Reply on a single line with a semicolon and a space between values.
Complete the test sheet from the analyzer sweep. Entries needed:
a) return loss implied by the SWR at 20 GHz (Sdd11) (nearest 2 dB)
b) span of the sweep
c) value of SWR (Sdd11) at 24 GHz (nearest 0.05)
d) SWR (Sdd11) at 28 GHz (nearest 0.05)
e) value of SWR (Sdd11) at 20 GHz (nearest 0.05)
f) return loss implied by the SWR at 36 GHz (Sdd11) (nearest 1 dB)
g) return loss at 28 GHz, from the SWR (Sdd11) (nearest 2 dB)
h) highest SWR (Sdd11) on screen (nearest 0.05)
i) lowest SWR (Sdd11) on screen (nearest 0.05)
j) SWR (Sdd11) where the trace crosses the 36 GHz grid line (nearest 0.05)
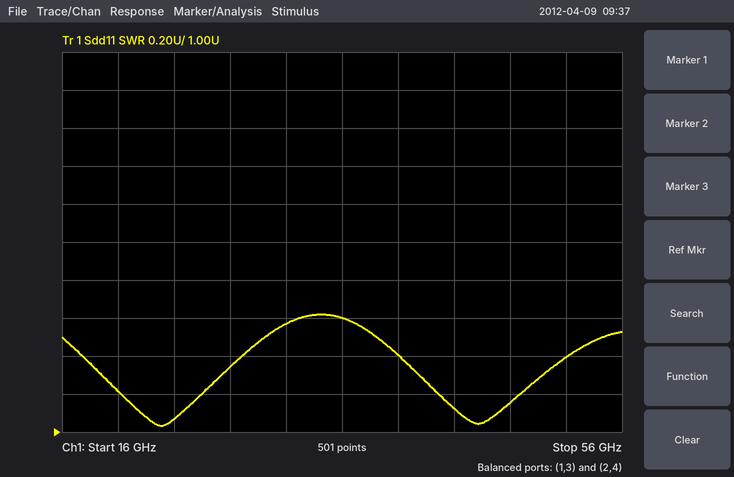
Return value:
20 dB; 40 GHz; 1.05; 1.35; 1.20; 13 dB; 16 dB; 1.60; 1.05; 1.60
